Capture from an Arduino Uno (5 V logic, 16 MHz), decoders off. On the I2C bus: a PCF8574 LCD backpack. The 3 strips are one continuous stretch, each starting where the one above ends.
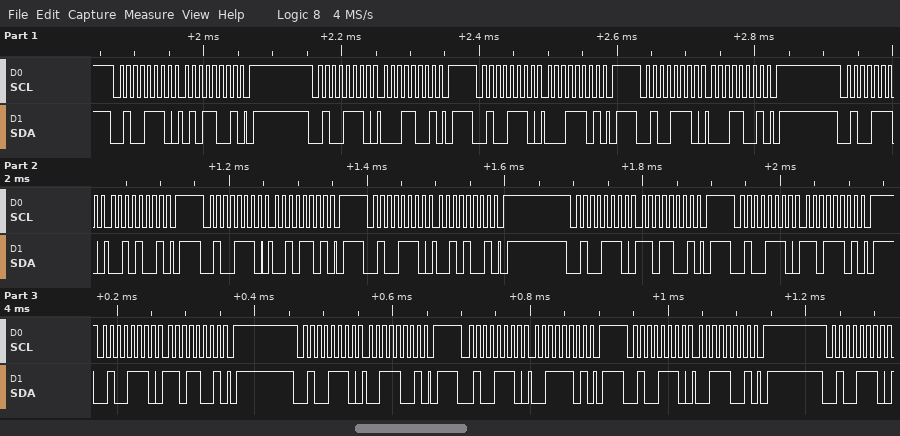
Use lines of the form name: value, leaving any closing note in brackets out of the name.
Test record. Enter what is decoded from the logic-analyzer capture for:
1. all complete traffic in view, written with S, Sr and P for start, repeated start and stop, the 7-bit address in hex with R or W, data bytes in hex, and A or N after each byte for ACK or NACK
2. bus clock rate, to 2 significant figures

all complete traffic in view, written with S, Sr and P for start, repeated start and stop, the 7-bit address in hex with R or W, data bytes in hex, and A or N after each byte for ACK or NACK: S 27W A 59 A P S 27W A 19 A P S 27W A 1D A P S 27W A 19 A P S 27W A 29 A P S 27W A 2D A P S 27W A 29 A P S 27W A D9 A P S 27W A DD A P S 27W A D9 A P S 27W A 39 A P S 27W A 3D A P S 27W A 39 A P S 27W A
bus clock rate, to 2 significant figures: 100 kHz
